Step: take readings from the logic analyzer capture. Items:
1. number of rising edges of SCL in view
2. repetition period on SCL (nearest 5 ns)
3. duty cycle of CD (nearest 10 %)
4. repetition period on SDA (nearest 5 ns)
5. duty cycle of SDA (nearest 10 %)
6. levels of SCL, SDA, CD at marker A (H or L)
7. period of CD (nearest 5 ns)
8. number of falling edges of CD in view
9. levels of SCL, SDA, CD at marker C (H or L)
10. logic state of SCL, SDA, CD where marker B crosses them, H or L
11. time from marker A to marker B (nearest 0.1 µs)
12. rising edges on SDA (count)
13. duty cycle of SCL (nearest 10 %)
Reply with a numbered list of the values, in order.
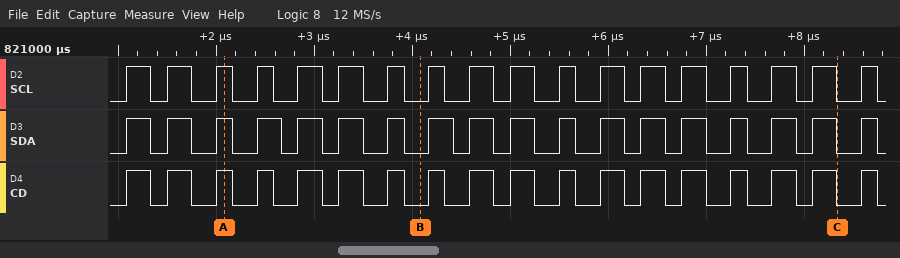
1. 18
2. 440 ns
3. 50 %
4. 440 ns
5. 50 %
6. SCL=H, SDA=H, CD=H
7. 440 ns
8. 18
9. SCL=L, SDA=L, CD=L
10. SCL=L, SDA=L, CD=L
11. 2 µs
12. 18
13. 50 %
